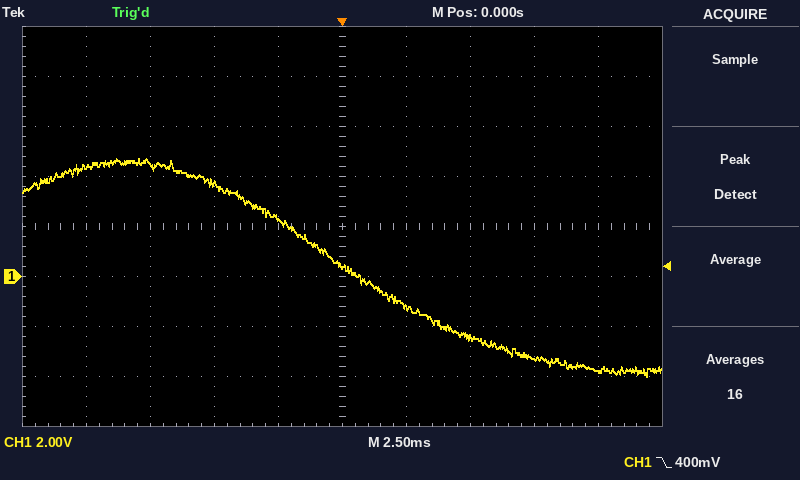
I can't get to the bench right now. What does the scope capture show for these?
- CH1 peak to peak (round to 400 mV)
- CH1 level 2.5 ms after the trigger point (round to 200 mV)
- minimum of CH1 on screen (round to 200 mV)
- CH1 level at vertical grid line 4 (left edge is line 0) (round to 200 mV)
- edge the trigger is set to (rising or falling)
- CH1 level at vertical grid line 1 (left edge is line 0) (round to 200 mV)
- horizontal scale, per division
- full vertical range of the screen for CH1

8.8 V
-1.2 V
-4.0 V
2.4 V
falling
4.4 V
2.5 ms
16 V
